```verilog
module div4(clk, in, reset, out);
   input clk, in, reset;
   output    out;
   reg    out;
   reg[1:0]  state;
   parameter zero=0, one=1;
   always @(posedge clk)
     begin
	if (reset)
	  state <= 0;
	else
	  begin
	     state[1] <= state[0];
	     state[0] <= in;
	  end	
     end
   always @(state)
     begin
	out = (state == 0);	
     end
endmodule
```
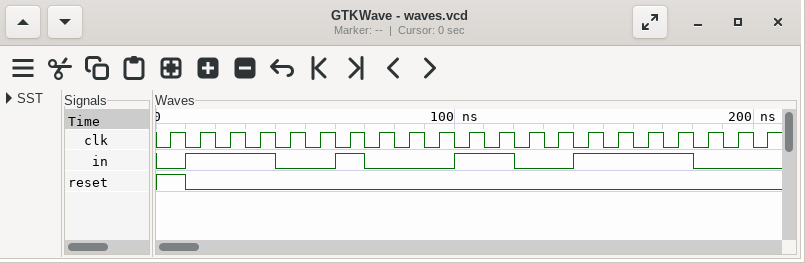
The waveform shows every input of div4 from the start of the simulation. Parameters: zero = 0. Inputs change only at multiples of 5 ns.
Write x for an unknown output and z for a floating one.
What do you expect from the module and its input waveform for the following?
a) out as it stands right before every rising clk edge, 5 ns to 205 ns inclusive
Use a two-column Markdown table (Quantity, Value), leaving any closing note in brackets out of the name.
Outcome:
| Quantity | Value |
|---|---|
| out as it stands right before every rising clk edge, 5 ns to 205 ns inclusive | x 1 0 0 0 0 1 0 0 1 1 0 0 0 1 0 0 0 0 0 1 |
